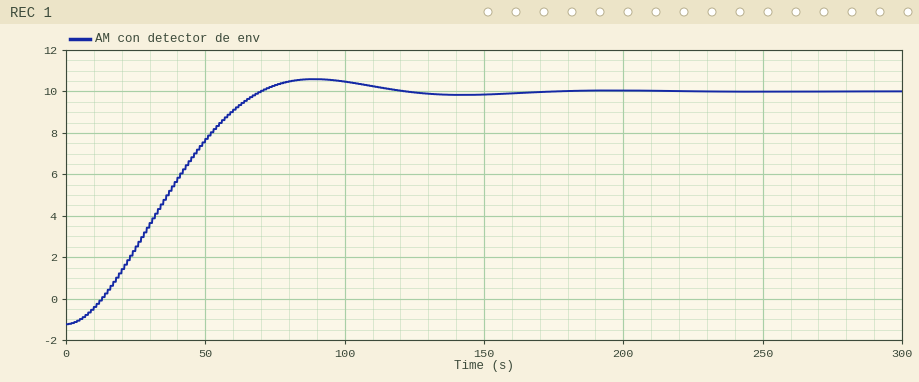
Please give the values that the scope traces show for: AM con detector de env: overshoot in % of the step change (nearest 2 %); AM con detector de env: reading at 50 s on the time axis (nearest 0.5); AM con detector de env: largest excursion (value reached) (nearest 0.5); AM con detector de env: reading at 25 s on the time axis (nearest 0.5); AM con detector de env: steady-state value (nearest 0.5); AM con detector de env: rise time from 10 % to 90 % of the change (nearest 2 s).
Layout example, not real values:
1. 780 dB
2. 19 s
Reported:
1. 6 %
2. 7.5
3. 10.5
4. 2.5
5. 10.0
6. 46 s
